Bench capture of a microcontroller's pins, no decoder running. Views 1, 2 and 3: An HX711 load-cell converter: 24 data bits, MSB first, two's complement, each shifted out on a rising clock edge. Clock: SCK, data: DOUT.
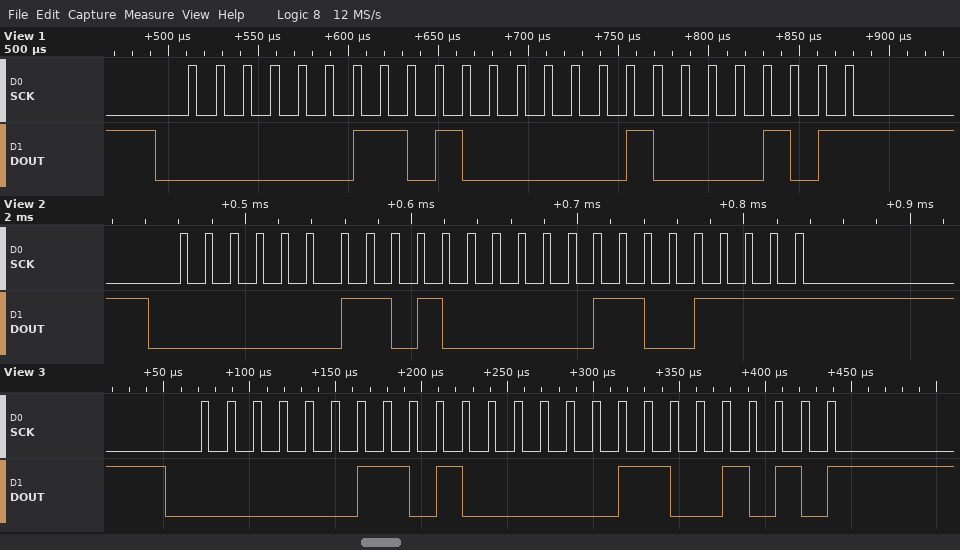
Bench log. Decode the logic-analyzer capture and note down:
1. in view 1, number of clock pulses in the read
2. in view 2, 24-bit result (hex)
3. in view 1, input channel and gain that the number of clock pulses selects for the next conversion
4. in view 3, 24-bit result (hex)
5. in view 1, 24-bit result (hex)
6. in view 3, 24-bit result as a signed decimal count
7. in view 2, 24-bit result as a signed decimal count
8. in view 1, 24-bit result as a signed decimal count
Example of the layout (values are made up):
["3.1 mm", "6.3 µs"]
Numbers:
["25", "0x0340CF", "channel A, gain 128", "0x0340CA", "0x034085", "213194", "213199", "213125"]
